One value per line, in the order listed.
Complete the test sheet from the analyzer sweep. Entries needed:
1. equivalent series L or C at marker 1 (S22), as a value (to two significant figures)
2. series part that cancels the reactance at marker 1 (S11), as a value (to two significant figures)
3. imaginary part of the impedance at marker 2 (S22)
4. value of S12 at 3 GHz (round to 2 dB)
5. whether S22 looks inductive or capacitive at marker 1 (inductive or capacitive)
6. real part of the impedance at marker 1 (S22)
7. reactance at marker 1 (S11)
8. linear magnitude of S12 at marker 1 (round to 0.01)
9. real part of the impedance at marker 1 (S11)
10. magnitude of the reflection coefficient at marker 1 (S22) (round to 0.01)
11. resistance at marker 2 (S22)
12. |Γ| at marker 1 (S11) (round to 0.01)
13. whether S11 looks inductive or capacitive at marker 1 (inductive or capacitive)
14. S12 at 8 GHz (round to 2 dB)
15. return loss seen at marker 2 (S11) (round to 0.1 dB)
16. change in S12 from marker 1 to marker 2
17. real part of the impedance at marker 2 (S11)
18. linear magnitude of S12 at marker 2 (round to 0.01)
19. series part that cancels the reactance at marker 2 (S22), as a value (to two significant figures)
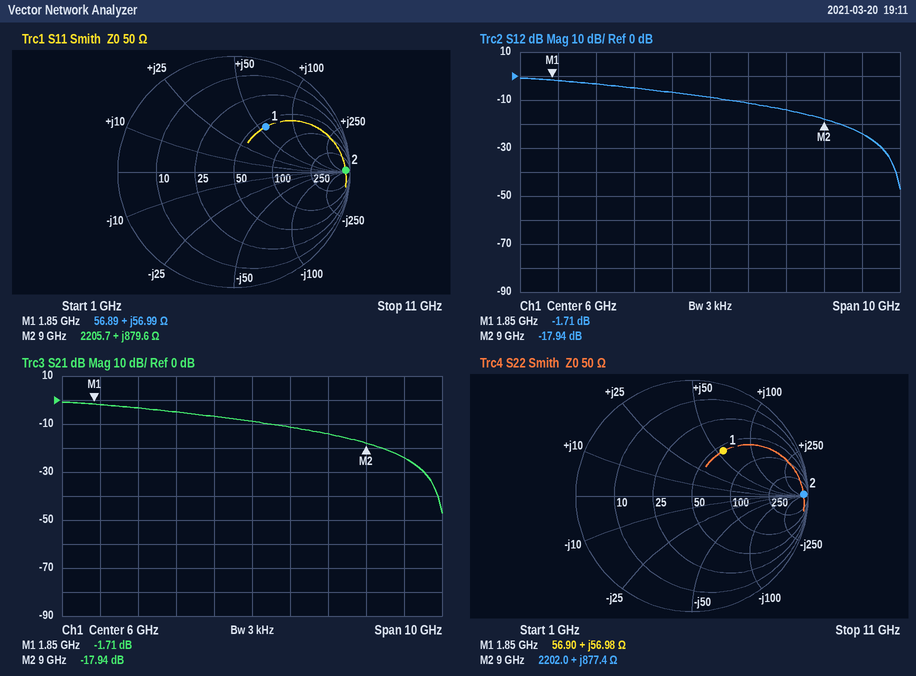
4.9 nH
1.5 pF
+877.4 Ω
-4 dB
inductive
56.90 Ω
+56.99 Ω
0.82
56.89 Ω
0.47
2202.0 Ω
0.47
inductive
-14 dB
0.3 dB
-16.23 dB
2205.7 Ω
0.13
20 fF
